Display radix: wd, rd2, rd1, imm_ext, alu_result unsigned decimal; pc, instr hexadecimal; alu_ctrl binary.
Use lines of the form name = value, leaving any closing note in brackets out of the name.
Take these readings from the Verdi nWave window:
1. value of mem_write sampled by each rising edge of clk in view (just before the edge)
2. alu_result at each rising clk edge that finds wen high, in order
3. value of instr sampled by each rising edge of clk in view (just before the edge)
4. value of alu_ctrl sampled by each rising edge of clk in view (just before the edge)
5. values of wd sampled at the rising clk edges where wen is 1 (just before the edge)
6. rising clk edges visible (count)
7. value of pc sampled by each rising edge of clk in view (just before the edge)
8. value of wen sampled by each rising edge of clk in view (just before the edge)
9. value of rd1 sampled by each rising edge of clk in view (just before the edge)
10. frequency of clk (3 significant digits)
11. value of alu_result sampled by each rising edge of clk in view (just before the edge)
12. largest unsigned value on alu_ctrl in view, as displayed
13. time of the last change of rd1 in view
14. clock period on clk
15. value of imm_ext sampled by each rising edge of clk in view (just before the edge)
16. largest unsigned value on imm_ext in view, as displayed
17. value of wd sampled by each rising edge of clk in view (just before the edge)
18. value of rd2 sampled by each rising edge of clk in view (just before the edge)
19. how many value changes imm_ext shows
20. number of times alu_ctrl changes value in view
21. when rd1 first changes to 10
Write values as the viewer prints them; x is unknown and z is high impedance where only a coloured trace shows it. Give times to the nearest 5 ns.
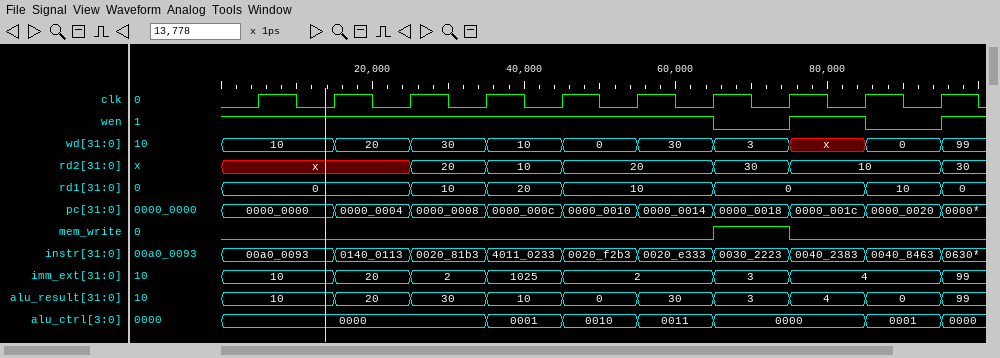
value of mem_write sampled by each rising edge of clk in view = 0 0 0 0 0 0 0 1 0 0
alu_result at each rising clk edge that finds wen high, in order = 10, 10, 20, 30, 10, 0, 30, 4
value of instr sampled by each rising edge of clk in view = 00a0_0093, 00a0_0093, 0140_0113, 0020_81b3, 4011_0233, 0020_f2b3, 0020_e333, 0030_2223, 0040_2383, 0040_8463
value of alu_ctrl sampled by each rising edge of clk in view = 0000, 0000, 0000, 0000, 0001, 0010, 0011, 0000, 0000, 0001
values of wd sampled at the rising clk edges where wen is 1 = 10, 10, 20, 30, 10, 0, 30, x
rising clk edges visible = 10
value of pc sampled by each rising edge of clk in view = 0000_0000, 0000_0000, 0000_0004, 0000_0008, 0000_000c, 0000_0010, 0000_0014, 0000_0018, 0000_001c, 0000_0020
value of wen sampled by each rising edge of clk in view = 1 1 1 1 1 1 1 0 1 0
value of rd1 sampled by each rising edge of clk in view = 0, 0, 0, 10, 20, 10, 10, 0, 0, 10
frequency of clk = 100 MHz
value of alu_result sampled by each rising edge of clk in view = 10, 10, 20, 30, 10, 0, 30, 3, 4, 0
largest unsigned value on alu_ctrl in view, as displayed = 0011
time of the last change of rd1 in view = 95 ns
clock period on clk = 10 ns
value of imm_ext sampled by each rising edge of clk in view = 10, 10, 20, 2, 1025, 2, 2, 3, 4, 4
largest unsigned value on imm_ext in view, as displayed = 1025
value of wd sampled by each rising edge of clk in view = 10, 10, 20, 30, 10, 0, 30, 3, x, 0
value of rd2 sampled by each rising edge of clk in view = x, x, x, 20, 10, 20, 20, 30, 10, 10
how many value changes imm_ext shows = 7
number of times alu_ctrl changes value in view = 6
when rd1 first changes to 10 = 25 ns
